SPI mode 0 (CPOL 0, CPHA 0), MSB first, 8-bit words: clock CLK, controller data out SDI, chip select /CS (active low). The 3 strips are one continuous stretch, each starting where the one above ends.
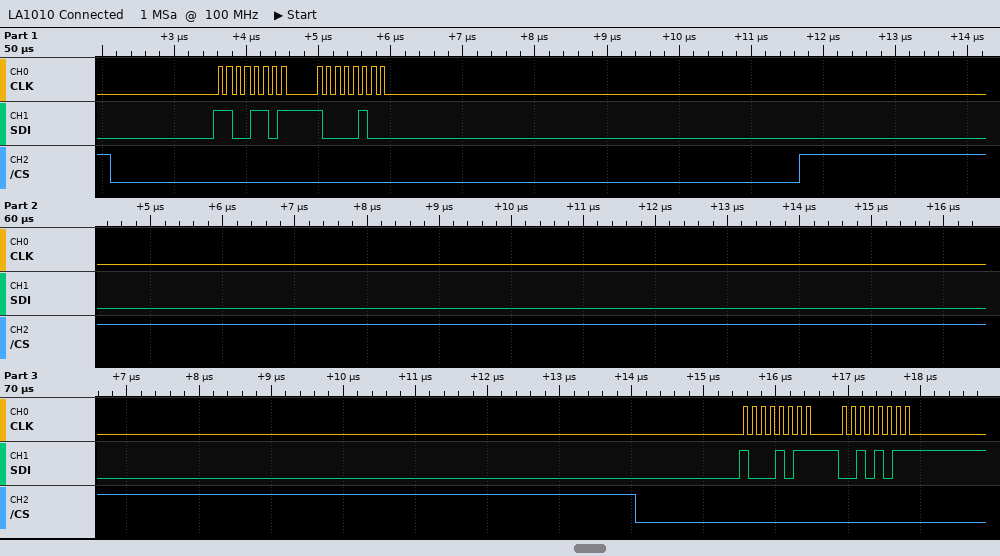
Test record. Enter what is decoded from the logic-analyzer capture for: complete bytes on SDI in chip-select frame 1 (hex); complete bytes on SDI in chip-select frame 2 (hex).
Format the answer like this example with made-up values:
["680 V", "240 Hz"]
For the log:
["CD 84", "8B 2B"]
